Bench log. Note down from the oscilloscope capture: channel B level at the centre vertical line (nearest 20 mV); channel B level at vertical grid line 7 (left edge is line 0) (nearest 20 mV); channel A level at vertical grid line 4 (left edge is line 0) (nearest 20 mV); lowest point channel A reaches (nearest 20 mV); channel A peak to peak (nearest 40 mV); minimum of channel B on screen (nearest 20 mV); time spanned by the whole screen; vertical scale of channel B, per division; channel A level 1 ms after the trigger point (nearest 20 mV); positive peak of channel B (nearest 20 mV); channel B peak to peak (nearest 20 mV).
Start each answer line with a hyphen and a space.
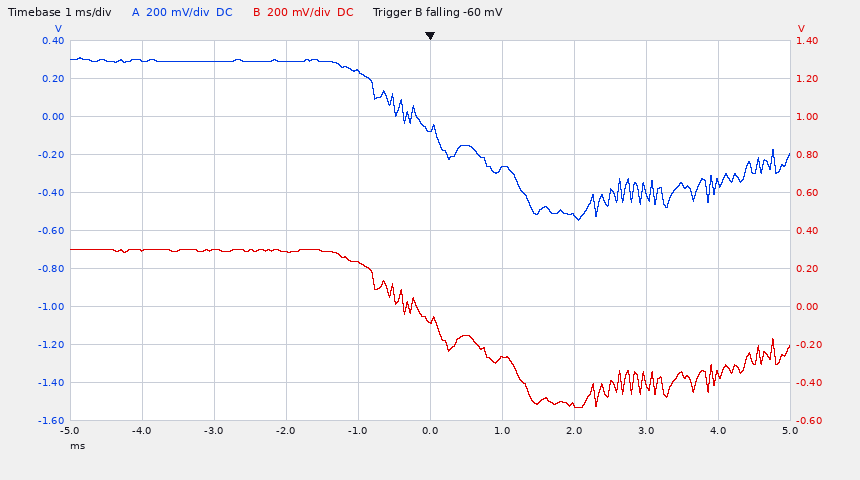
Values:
- -80 mV
- -520 mV
- 240 mV
- -540 mV
- 840 mV
- -540 mV
- 10 ms
- 200 mV
- -280 mV
- 300 mV
- 840 mV
